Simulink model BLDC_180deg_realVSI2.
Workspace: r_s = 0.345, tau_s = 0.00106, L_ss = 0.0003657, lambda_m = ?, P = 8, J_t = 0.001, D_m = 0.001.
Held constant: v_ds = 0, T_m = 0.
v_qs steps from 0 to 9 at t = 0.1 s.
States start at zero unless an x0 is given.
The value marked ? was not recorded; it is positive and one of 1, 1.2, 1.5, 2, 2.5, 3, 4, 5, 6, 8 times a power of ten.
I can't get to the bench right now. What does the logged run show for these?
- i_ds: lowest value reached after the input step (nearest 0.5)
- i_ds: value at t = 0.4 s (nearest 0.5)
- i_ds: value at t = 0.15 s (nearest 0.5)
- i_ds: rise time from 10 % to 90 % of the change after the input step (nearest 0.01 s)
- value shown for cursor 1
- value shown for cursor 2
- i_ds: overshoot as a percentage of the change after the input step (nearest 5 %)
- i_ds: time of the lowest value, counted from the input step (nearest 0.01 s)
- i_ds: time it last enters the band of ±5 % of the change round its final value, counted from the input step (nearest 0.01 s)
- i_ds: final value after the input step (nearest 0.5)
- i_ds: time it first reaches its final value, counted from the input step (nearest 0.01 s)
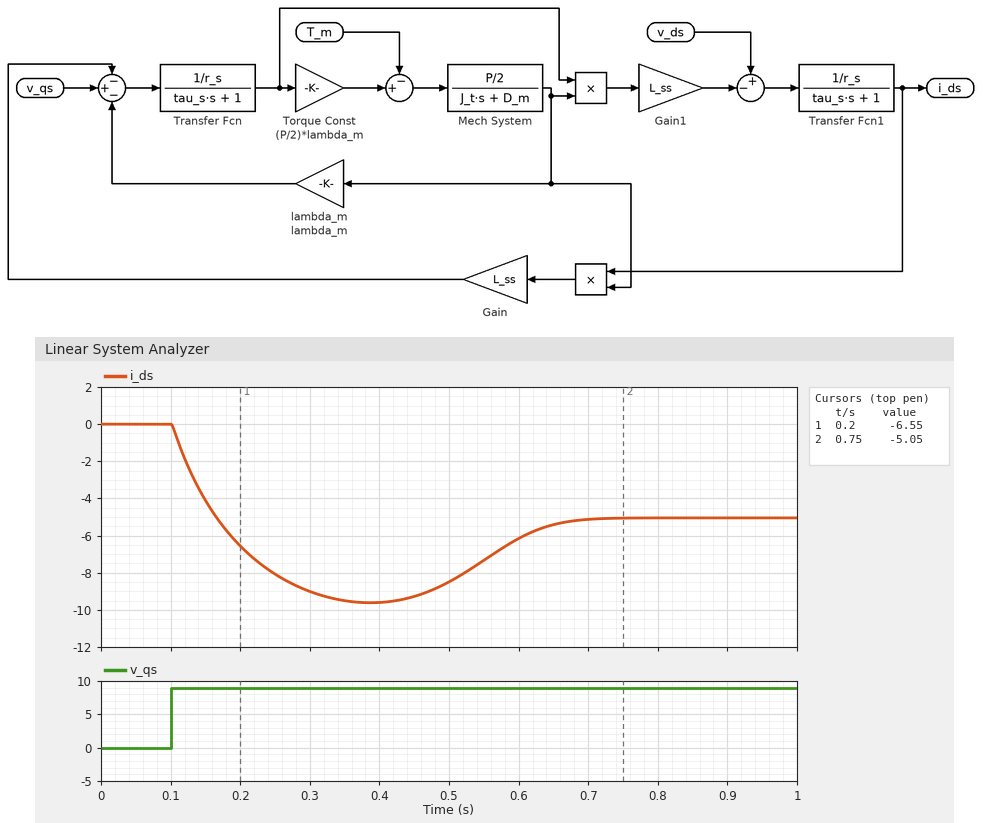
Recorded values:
-9.5
-9.5
-4.0
0.05 s
-6.55
-5.05
90 %
0.29 s
0.56 s
-5.0
0.07 s
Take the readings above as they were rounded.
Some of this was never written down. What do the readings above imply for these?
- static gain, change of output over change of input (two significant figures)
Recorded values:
-0.56
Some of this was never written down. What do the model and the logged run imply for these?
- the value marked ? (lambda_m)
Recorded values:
0.01
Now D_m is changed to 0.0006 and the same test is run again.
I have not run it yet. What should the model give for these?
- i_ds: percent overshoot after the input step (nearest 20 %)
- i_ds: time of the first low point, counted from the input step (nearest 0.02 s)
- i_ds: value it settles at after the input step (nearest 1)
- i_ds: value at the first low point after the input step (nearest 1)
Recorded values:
200 %
0.26 s
-3
-10
